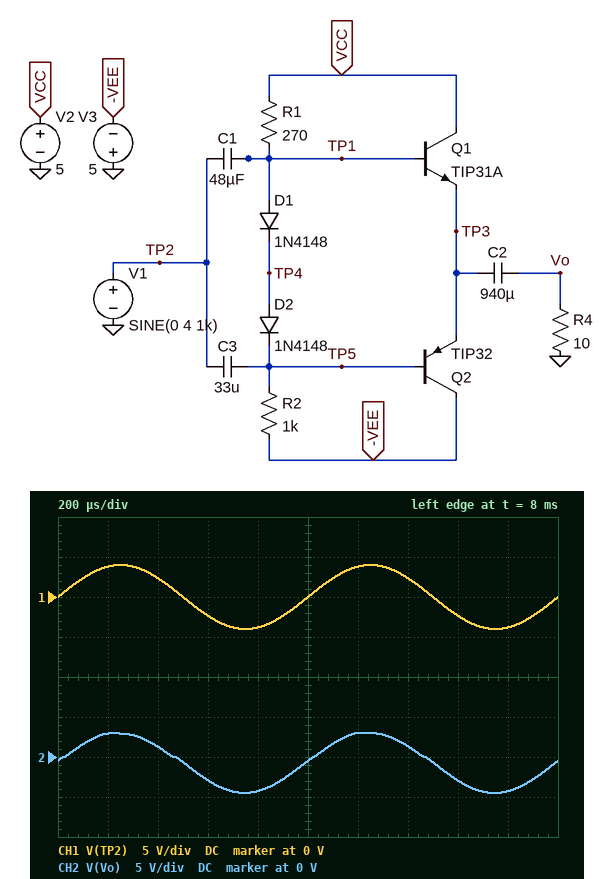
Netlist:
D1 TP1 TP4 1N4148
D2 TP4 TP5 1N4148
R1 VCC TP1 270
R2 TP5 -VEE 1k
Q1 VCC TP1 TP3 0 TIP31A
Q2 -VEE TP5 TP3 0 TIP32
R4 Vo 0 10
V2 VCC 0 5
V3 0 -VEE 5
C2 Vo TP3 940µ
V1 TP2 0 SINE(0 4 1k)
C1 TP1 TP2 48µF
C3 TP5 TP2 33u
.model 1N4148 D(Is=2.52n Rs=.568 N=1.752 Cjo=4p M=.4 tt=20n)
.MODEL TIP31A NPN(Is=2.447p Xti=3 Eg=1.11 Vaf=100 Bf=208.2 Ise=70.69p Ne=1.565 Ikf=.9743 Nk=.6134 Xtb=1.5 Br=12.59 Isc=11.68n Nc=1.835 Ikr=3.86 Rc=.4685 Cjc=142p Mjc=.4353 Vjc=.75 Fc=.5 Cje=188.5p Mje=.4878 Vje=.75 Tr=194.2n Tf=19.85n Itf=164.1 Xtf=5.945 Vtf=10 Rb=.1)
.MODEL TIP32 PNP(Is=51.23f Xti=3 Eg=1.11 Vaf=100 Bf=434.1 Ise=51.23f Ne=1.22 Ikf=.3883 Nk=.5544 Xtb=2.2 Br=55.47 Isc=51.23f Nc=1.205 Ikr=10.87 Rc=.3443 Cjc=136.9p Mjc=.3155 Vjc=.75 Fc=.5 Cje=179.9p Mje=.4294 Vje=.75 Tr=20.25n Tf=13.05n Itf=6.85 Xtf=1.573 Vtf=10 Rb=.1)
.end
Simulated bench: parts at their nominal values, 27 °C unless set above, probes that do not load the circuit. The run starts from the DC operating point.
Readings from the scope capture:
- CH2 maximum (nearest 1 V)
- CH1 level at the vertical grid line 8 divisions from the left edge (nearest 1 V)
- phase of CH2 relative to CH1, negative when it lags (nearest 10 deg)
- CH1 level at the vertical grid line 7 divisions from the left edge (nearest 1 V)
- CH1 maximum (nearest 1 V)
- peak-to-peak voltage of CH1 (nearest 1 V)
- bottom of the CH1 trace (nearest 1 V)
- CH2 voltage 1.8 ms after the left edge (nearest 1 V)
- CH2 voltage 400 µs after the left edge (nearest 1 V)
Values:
3 V
-2 V
0 deg
2 V
4 V
8 V
-4 V
-4 V
1 V
